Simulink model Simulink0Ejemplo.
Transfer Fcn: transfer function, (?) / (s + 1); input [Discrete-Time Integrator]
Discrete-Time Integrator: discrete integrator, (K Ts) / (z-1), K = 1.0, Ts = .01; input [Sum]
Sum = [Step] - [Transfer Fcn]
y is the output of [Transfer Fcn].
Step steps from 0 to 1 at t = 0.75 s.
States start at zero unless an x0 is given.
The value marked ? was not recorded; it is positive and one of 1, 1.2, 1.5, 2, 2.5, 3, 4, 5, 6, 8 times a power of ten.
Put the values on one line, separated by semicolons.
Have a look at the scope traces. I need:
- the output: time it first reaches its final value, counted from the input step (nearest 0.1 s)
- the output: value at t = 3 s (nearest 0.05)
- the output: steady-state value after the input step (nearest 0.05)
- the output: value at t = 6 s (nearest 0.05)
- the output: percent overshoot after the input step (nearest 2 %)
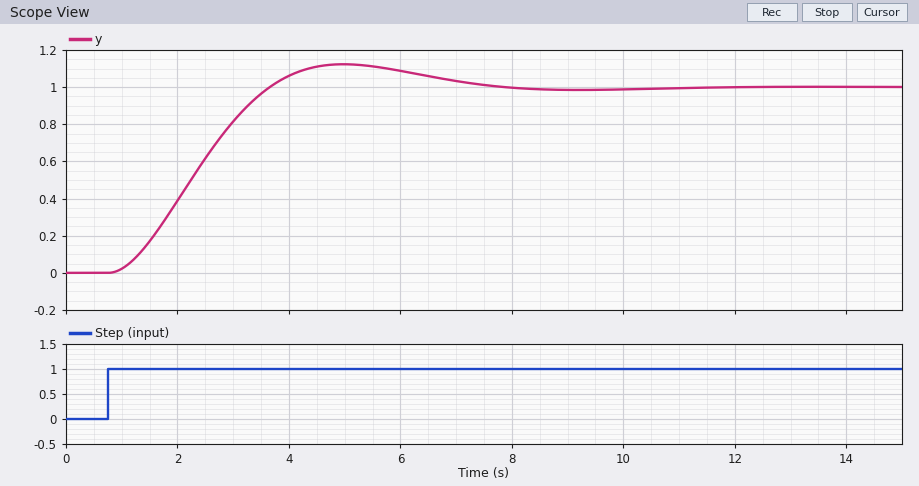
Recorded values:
2.9 s; 0.80; 1.00; 1.10; 12 %
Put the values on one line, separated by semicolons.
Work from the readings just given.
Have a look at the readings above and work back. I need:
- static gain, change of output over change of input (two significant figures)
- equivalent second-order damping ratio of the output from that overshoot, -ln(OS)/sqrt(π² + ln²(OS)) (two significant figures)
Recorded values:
1.0; 0.56
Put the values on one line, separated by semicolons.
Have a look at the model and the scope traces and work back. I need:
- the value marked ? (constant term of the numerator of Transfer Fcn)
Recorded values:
0.8
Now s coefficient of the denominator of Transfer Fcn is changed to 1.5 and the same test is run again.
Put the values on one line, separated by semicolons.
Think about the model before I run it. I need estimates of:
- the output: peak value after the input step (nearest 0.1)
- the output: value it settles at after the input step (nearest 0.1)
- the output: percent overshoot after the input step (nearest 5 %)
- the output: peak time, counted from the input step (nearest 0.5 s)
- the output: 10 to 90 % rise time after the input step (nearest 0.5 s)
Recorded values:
1.2; 1.0; 20 %; 5.0 s; 2.0 s
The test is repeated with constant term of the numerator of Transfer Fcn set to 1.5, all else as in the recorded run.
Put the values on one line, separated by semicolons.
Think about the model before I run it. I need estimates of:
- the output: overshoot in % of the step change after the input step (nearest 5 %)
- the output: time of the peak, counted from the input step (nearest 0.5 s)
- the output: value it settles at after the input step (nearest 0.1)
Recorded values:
25 %; 3.0 s; 1.0
